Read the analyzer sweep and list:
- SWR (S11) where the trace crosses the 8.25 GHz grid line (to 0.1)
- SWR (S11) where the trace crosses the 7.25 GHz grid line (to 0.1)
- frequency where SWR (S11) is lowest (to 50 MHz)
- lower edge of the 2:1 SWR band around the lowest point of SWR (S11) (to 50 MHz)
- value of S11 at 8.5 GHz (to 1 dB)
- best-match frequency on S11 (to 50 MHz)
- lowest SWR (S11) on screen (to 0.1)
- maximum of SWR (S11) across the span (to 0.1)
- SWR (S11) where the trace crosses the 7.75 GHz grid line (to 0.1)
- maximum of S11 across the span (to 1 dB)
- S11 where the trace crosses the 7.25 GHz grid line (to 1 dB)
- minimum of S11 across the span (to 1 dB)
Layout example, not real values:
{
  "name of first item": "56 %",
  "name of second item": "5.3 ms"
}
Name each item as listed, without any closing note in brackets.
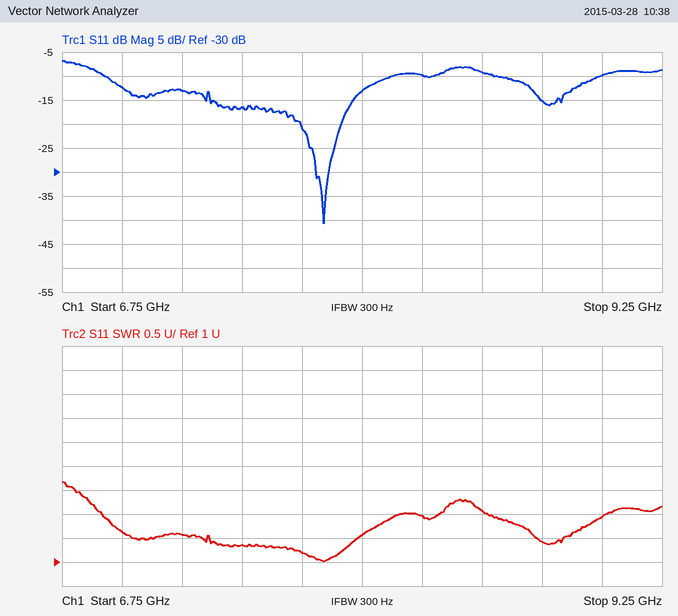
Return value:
{
  "SWR (S11) where the trace crosses the 8.25 GHz grid line": "2.0",
  "SWR (S11) where the trace crosses the 7.25 GHz grid line": "1.6",
  "frequency where SWR (S11) is lowest": "7.85 GHz",
  "lower edge of the 2:1 SWR band around the lowest point of SWR (S11)": "6.90 GHz",
  "value of S11 at 8.5 GHz": "-9 dB",
  "best-match frequency on S11": "7.85 GHz",
  "lowest SWR (S11) on screen": "1.0",
  "maximum of SWR (S11) across the span": "2.7",
  "SWR (S11) where the trace crosses the 7.75 GHz grid line": "1.2",
  "maximum of S11 across the span": "-7 dB",
  "S11 where the trace crosses the 7.25 GHz grid line": "-13 dB",
  "minimum of S11 across the span": "-41 dB"
}
